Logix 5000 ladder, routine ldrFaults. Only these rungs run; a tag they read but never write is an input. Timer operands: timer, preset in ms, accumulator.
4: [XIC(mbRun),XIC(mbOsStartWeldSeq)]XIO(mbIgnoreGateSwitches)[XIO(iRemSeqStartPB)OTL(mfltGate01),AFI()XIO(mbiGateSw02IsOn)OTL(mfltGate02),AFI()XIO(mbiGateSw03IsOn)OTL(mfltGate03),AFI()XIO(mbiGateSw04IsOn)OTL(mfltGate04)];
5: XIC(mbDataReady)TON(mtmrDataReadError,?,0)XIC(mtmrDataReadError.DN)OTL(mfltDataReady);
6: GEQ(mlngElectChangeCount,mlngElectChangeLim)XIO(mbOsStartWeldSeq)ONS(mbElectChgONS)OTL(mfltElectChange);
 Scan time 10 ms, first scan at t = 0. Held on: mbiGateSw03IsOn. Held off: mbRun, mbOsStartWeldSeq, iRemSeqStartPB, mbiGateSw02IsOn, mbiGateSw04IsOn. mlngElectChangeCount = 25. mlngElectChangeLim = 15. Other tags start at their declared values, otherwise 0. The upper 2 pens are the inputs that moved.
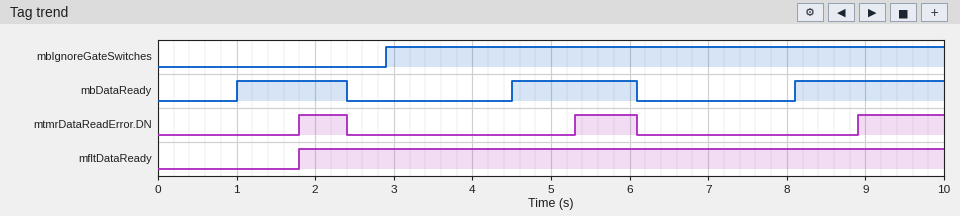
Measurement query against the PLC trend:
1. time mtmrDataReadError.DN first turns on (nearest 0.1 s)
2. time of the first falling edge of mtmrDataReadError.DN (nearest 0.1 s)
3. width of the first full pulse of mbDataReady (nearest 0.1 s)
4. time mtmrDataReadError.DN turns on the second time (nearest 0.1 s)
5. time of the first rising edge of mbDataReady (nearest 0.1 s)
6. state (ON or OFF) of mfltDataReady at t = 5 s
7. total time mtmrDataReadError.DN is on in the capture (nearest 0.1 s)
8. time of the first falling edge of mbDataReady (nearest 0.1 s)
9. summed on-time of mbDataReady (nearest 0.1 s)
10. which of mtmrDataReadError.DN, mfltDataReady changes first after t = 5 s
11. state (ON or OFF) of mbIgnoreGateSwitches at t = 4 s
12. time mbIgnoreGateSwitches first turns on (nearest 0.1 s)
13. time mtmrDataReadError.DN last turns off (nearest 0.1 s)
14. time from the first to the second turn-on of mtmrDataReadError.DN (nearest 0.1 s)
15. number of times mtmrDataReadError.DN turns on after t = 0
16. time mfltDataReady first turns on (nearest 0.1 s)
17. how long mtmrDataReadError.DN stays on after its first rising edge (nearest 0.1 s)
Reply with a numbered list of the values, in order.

1. 1.8 s
2. 2.4 s
3. 1.4 s
4. 5.3 s
5. 1.0 s
6. ON
7. 2.5 s
8. 2.4 s
9. 4.9 s
10. mtmrDataReadError.DN
11. ON
12. 2.9 s
13. 6.1 s
14. 3.5 s
15. 3
16. 1.8 s
17. 0.6 s
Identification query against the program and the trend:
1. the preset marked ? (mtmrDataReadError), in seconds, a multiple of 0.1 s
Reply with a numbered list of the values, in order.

1. 0.8 s
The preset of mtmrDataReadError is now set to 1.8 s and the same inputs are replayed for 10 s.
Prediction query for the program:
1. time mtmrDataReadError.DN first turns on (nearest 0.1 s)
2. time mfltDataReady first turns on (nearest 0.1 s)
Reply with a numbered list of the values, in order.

1. 9.9 s
2. 9.9 s
